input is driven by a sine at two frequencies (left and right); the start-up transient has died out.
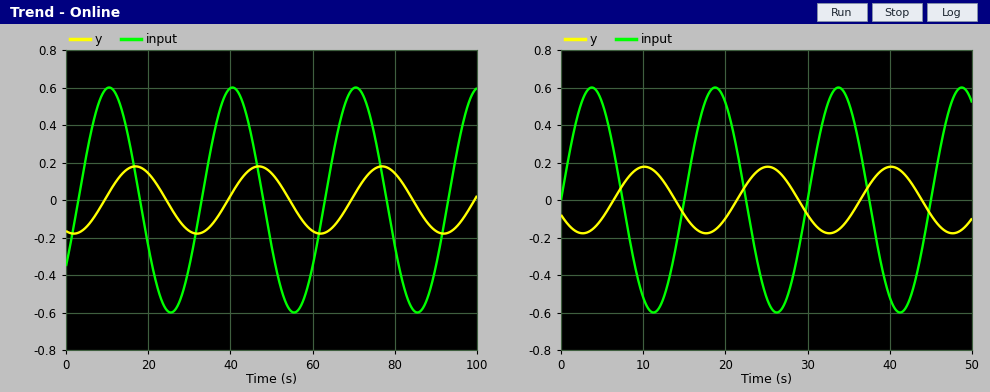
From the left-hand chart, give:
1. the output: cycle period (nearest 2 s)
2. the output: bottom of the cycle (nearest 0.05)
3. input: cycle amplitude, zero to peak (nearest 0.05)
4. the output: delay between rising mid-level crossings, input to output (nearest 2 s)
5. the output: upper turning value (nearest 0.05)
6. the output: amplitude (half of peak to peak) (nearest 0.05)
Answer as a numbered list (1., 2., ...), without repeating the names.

1. 30 s
2. -0.20
3. 0.60
4. 6 s
5. 0.20
6. 0.20
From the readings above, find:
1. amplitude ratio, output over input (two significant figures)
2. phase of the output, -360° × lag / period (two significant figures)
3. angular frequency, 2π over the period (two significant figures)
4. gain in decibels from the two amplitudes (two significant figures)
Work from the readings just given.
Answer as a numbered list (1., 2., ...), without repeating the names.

1. 0.33
2. -72°
3. 0.21 rad/s
4. -9.5 dB
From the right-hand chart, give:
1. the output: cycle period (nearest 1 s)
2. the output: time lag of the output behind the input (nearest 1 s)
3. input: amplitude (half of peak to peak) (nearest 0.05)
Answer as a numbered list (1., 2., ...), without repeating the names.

1. 15 s
2. 6 s
3. 0.60
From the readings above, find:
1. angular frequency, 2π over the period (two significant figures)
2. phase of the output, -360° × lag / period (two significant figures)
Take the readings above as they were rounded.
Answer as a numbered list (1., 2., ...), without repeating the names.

1. 0.42 rad/s
2. -140°
